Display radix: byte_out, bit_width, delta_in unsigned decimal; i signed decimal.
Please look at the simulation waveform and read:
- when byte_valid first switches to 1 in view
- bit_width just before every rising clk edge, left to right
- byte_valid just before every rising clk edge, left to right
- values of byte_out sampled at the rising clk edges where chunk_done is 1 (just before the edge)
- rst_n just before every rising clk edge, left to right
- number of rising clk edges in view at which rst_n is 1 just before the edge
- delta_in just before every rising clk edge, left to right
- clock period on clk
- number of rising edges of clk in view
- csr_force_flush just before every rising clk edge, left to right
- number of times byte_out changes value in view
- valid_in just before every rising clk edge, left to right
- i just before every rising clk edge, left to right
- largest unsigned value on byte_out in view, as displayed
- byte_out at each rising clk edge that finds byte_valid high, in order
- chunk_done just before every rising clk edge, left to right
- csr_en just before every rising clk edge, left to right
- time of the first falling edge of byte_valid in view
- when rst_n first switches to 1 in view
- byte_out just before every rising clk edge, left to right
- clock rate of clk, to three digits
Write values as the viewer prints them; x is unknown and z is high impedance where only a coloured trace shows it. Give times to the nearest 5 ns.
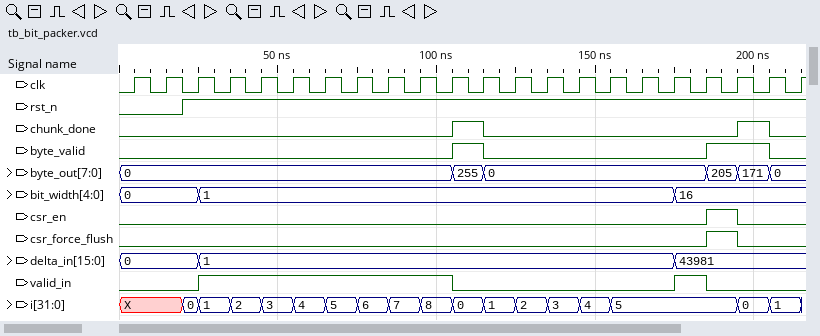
105 ns
0, 0, 0, 1, 1, 1, 1, 1, 1, 1, 1, 1, 1, 1, 1, 1, 1, 1, 16, 16, 16, 16
0 0 0 0 0 0 0 0 0 0 0 1 0 0 0 0 0 0 0 1 1 0
255, 171
0 0 1 1 1 1 1 1 1 1 1 1 1 1 1 1 1 1 1 1 1 1
20
0, 0, 0, 1, 1, 1, 1, 1, 1, 1, 1, 1, 1, 1, 1, 1, 1, 1, 43981, 43981, 43981, 43981
10 ns
22
0 0 0 0 0 0 0 0 0 0 0 0 0 0 0 0 0 0 0 1 0 0
5
0 0 0 1 1 1 1 1 1 1 1 0 0 0 0 0 0 0 1 0 0 0
X, X, 0, 1, 2, 3, 4, 5, 6, 7, 8, 0, 1, 2, 3, 4, 5, 5, 5, 5, 0, 1
255
255, 205, 171
0 0 0 0 0 0 0 0 0 0 0 1 0 0 0 0 0 0 0 0 1 0
0 0 0 0 0 0 0 0 0 0 0 0 0 0 0 0 0 0 0 1 0 0
115 ns
20 ns
0, 0, 0, 0, 0, 0, 0, 0, 0, 0, 0, 255, 0, 0, 0, 0, 0, 0, 0, 205, 171, 0
100 MHz
